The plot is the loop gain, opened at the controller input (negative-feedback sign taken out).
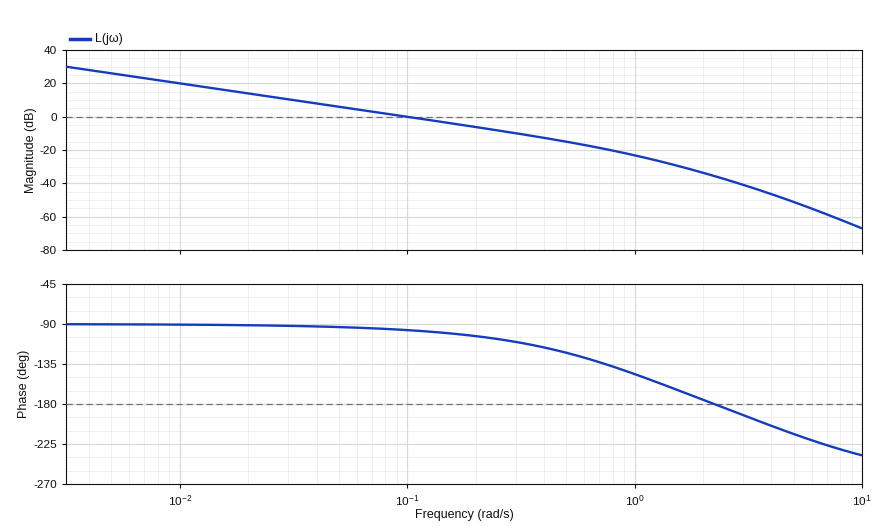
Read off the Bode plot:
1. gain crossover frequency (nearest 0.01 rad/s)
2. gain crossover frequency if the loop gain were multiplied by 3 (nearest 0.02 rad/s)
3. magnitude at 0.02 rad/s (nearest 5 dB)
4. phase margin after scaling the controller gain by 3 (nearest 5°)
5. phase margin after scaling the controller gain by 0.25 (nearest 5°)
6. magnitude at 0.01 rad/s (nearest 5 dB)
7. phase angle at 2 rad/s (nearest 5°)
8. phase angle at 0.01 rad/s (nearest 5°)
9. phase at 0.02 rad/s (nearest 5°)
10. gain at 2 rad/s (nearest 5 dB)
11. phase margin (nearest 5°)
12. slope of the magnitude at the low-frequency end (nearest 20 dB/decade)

0.10 rad/s
0.28 rad/s
15 dB
70°
90°
20 dB
-175°
-90°
-90°
-35 dB
85°
-20 dB/decade
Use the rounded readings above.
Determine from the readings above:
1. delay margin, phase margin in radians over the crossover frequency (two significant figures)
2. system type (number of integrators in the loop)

15 s
1
